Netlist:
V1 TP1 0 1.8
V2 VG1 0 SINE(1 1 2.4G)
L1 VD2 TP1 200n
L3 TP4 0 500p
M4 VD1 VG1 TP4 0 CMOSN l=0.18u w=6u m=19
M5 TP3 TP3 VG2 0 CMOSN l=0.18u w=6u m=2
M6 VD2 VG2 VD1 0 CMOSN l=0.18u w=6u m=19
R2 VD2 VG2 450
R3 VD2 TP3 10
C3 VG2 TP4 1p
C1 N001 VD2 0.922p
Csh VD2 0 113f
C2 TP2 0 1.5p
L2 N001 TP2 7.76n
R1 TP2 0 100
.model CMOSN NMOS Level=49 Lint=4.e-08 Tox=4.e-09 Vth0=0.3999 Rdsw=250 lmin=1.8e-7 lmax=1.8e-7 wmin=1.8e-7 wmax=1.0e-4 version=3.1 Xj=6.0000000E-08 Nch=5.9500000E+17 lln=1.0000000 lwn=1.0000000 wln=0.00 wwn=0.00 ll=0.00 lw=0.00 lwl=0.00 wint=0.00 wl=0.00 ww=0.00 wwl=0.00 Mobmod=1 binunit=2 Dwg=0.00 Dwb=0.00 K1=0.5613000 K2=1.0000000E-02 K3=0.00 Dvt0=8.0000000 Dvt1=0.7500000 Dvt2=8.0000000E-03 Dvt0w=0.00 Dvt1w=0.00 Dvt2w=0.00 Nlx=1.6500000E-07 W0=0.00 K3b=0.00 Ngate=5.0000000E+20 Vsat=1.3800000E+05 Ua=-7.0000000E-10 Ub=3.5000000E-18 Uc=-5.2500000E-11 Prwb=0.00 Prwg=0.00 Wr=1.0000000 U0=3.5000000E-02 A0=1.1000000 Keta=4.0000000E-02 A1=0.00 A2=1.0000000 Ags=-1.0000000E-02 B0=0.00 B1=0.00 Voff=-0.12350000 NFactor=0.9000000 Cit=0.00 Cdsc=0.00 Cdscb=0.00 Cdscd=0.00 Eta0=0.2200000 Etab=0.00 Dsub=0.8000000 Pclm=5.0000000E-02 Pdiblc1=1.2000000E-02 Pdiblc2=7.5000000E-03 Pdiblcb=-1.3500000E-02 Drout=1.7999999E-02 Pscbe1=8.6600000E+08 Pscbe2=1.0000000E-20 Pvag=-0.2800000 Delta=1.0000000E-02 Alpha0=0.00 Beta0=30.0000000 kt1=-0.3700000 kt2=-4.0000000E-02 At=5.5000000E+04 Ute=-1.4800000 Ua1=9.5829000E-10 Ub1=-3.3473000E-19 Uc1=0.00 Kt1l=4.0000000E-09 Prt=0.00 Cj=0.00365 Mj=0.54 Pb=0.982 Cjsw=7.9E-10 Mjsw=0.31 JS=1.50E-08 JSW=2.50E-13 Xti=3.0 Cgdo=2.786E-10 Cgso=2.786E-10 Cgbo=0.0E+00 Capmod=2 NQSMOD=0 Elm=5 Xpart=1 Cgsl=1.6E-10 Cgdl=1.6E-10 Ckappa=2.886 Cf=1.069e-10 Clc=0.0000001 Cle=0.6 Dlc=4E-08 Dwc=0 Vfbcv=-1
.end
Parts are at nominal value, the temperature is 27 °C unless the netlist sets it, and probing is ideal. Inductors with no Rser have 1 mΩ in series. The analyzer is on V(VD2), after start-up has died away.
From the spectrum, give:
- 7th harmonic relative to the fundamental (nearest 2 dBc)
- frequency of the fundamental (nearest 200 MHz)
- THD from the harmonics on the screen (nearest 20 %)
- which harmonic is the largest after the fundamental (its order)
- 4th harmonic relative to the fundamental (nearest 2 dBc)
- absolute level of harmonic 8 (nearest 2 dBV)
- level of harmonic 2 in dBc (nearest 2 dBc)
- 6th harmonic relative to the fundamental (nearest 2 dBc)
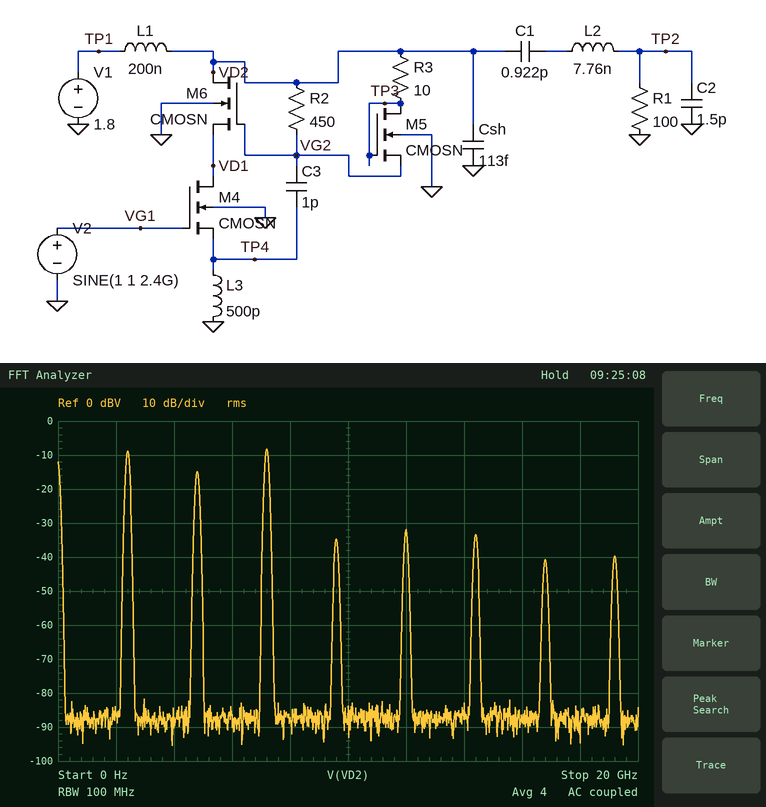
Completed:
-32 dBc
2.4 GHz
120 %
3
-26 dBc
-40 dBV
-6 dBc
-24 dBc
